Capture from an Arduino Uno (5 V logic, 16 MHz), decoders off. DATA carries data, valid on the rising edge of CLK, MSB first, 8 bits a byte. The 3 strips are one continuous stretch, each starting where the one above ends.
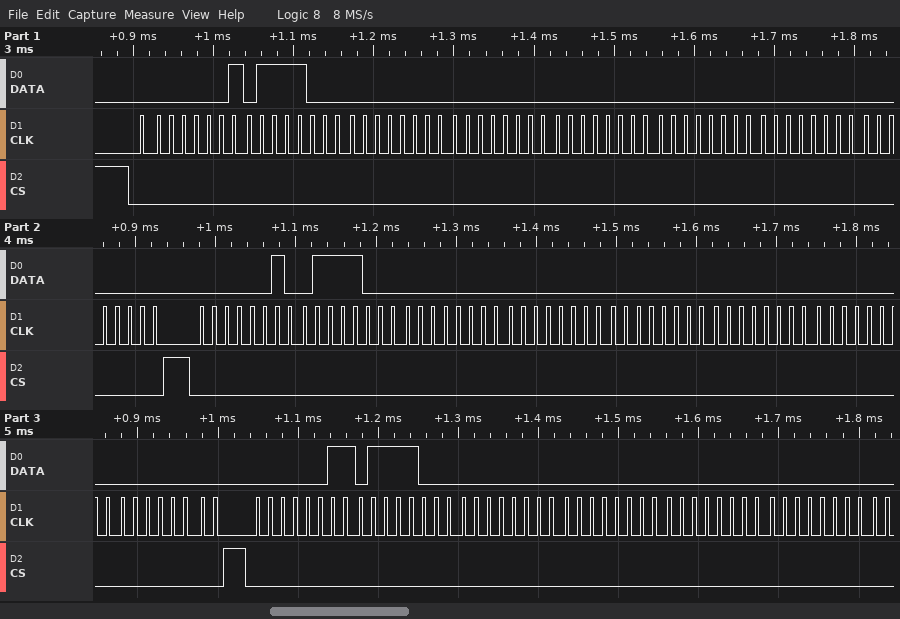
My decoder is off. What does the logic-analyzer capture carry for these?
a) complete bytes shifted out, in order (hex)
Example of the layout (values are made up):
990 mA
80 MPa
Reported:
01 78 00 00 00 00 00 00 02 78 00 00 00 00 00 00 03 78 00 00 00 00
